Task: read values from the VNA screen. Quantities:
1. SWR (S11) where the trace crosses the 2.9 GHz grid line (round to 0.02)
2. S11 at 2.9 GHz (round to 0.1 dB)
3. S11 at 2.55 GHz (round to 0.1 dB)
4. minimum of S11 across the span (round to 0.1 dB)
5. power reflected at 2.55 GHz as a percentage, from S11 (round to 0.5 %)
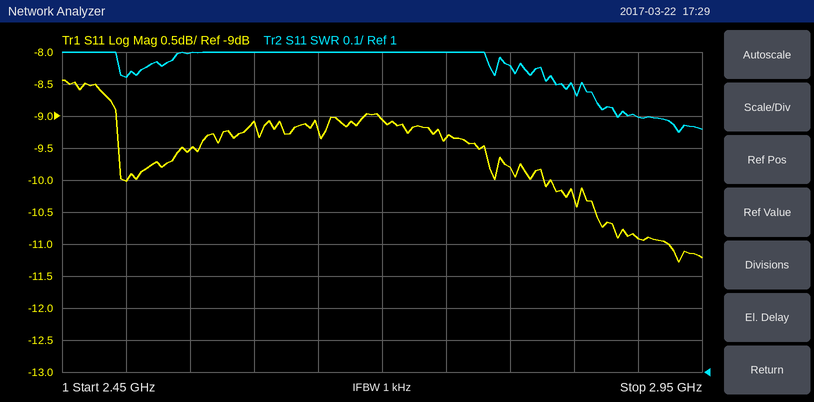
1.80
-10.9 dB
-9.5 dB
-11.3 dB
11.0 %
